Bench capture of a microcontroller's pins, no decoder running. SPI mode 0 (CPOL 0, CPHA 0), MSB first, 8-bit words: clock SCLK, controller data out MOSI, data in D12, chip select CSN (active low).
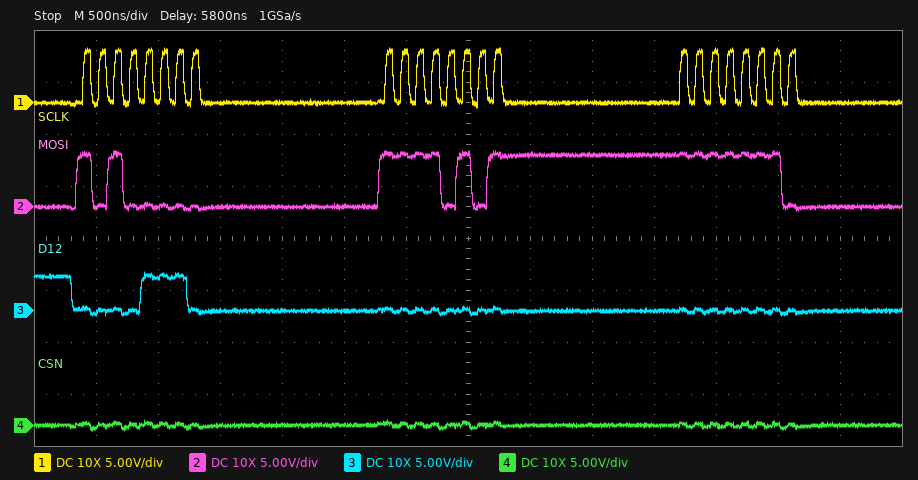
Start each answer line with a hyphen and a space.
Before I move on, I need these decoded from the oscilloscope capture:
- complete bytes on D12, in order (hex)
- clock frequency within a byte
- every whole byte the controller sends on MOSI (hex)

- 0E 00 00
- 8 MHz
- A0 F5 FE
